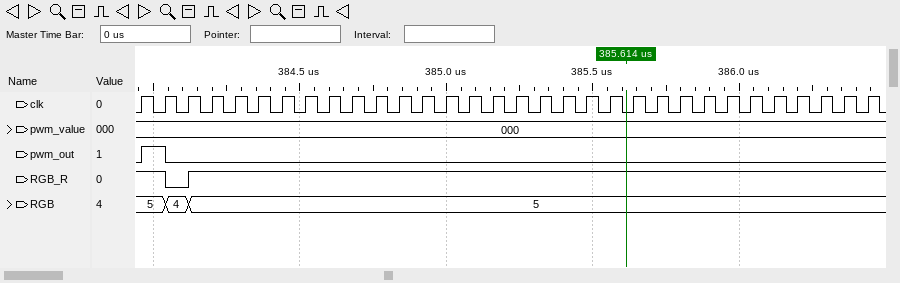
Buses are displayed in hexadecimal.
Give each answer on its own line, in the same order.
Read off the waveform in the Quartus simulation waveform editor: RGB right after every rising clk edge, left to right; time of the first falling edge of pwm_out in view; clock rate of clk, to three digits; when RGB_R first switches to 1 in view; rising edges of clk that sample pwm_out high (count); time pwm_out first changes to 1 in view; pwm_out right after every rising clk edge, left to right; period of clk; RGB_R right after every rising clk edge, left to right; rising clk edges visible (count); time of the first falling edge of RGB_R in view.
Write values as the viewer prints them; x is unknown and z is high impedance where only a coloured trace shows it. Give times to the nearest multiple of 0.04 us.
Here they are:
5, 4, 5, 5, 5, 5, 5, 5, 5, 5, 5, 5, 5, 5, 5, 5, 5, 5, 5, 5, 5, 5, 5, 5, 5, 5, 5, 5, 5, 5, 5, 5
384.04 us
12.5 MHz
384.12 us
1
383.96 us
1 0 0 0 0 0 0 0 0 0 0 0 0 0 0 0 0 0 0 0 0 0 0 0 0 0 0 0 0 0 0 0
0.08 us
1 0 1 1 1 1 1 1 1 1 1 1 1 1 1 1 1 1 1 1 1 1 1 1 1 1 1 1 1 1 1 1
32
384.04 us
